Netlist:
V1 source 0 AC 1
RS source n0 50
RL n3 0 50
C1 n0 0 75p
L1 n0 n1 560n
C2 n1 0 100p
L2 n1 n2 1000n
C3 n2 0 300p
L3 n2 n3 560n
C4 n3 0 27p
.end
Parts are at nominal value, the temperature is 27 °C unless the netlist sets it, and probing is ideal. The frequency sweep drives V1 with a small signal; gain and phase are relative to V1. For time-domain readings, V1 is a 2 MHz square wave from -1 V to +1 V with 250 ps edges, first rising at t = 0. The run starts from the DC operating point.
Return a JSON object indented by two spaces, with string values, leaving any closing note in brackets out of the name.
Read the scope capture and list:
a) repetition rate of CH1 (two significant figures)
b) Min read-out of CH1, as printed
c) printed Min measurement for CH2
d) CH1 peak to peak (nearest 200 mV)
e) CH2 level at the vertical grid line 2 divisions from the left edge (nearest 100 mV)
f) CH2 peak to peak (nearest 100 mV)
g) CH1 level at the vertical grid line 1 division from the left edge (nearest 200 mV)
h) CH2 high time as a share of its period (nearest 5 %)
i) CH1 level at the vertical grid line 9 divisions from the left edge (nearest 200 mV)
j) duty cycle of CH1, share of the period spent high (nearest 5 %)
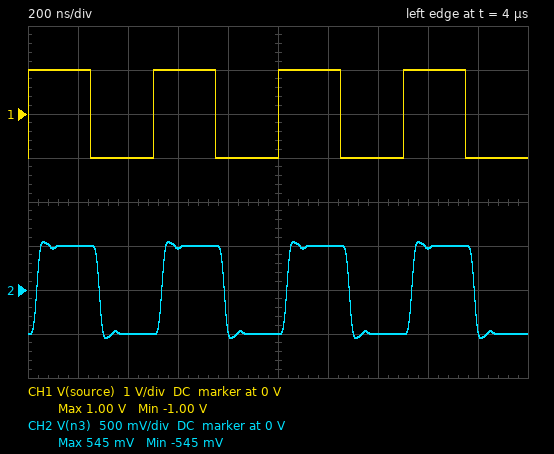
{
  "repetition rate of CH1": "2.0 MHz",
  "Min read-out of CH1, as printed": "-1.00 V",
  "printed Min measurement for CH2": "-545 mV",
  "CH1 peak to peak": "2.0 V",
  "CH2 level at the vertical grid line 2 divisions from the left edge": "-500 mV",
  "CH2 peak to peak": "1.1 V",
  "CH1 level at the vertical grid line 1 division from the left edge": "1.0 V",
  "CH2 high time as a share of its period": "50 %",
  "CH1 level at the vertical grid line 9 divisions from the left edge": "-1.0 V",
  "duty cycle of CH1, share of the period spent high": "50 %"
}
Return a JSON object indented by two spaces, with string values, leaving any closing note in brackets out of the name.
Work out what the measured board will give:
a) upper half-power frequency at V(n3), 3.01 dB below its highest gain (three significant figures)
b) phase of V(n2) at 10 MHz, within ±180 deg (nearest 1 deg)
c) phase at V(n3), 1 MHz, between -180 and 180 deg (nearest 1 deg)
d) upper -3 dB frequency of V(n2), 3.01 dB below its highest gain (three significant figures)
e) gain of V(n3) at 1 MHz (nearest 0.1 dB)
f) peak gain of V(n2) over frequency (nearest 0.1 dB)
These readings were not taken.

{
  "upper half-power frequency at V(n3), 3.01 dB below its highest gain": "15.3 MHz",
  "phase of V(n2) at 10 MHz, within ±180 deg": "-87 deg",
  "phase at V(n3), 1 MHz, between -180 and 180 deg": "-12 deg",
  "upper -3 dB frequency of V(n2), 3.01 dB below its highest gain": "18.4 MHz",
  "gain of V(n3) at 1 MHz": "-6.0 dB",
  "peak gain of V(n2) over frequency": "-5.1 dB"
}
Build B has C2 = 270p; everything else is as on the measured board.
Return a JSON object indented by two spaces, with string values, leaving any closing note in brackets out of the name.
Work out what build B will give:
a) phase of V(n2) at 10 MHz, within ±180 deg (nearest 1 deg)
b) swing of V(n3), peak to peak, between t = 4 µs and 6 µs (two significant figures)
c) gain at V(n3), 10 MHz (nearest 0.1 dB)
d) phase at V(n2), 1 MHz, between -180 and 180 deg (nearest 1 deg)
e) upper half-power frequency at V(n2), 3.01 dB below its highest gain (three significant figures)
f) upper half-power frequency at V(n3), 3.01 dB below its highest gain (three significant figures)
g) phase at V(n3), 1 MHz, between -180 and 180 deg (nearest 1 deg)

{
  "phase of V(n2) at 10 MHz, within ±180 deg": "-105 deg",
  "swing of V(n3), peak to peak, between t = 4 µs and 6 µs": "1.3 V",
  "gain at V(n3), 10 MHz": "-6.0 dB",
  "phase at V(n2), 1 MHz, between -180 and 180 deg": "-10 deg",
  "upper half-power frequency at V(n2), 3.01 dB below its highest gain": "18.6 MHz",
  "upper half-power frequency at V(n3), 3.01 dB below its highest gain": "17.9 MHz",
  "phase at V(n3), 1 MHz, between -180 and 180 deg": "-14 deg"
}
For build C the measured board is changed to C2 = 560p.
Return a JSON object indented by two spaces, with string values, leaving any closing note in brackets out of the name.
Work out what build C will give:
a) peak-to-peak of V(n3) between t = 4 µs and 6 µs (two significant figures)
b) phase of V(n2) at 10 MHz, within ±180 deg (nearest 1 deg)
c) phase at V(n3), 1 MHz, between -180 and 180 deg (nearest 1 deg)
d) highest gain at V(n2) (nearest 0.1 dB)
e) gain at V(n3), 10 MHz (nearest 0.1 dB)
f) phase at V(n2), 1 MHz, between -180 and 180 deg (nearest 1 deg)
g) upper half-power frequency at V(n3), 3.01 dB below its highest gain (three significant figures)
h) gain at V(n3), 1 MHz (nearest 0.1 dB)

{
  "peak-to-peak of V(n3) between t = 4 µs and 6 µs": "1.2 V",
  "phase of V(n2) at 10 MHz, within ±180 deg": "-136 deg",
  "phase at V(n3), 1 MHz, between -180 and 180 deg": "-16 deg",
  "highest gain at V(n2)": "-5.7 dB",
  "gain at V(n3), 10 MHz": "-7.1 dB",
  "phase at V(n2), 1 MHz, between -180 and 180 deg": "-12 deg",
  "upper half-power frequency at V(n3), 3.01 dB below its highest gain": "13.9 MHz",
  "gain at V(n3), 1 MHz": "-6.0 dB"
}
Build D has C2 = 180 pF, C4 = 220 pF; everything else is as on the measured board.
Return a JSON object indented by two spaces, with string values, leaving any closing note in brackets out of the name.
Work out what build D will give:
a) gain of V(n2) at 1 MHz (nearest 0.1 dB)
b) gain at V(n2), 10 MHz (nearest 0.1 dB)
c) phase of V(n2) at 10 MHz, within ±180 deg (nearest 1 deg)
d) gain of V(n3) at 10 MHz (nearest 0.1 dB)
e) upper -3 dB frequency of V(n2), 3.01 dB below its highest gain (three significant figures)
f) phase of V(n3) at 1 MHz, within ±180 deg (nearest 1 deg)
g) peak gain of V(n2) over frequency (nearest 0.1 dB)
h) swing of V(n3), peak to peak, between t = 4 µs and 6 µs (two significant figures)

{
  "gain of V(n2) at 1 MHz": "-6.0 dB",
  "gain at V(n2), 10 MHz": "-8.3 dB",
  "phase of V(n2) at 10 MHz, within ±180 deg": "-94 deg",
  "gain of V(n3) at 10 MHz": "-7.1 dB",
  "upper -3 dB frequency of V(n2), 3.01 dB below its highest gain": "22.5 MHz",
  "phase of V(n3) at 1 MHz, within ±180 deg": "-15 deg",
  "peak gain of V(n2) over frequency": "-3.1 dB",
  "swing of V(n3), peak to peak, between t = 4 µs and 6 µs": "1.2 V"
}
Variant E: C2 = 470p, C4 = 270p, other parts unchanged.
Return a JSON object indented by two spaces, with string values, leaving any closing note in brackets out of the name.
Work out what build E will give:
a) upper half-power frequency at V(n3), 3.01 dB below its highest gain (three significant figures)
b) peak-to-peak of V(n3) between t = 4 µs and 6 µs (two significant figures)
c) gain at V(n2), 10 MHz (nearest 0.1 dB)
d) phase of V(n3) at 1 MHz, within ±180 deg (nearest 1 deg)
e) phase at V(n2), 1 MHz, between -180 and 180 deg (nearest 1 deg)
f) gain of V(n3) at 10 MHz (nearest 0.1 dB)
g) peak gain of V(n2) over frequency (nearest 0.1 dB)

{
  "upper half-power frequency at V(n3), 3.01 dB below its highest gain": "12.3 MHz",
  "peak-to-peak of V(n3) between t = 4 µs and 6 µs": "1.2 V",
  "gain at V(n2), 10 MHz": "-8.8 dB",
  "phase of V(n3) at 1 MHz, within ±180 deg": "-18 deg",
  "phase at V(n2), 1 MHz, between -180 and 180 deg": "-14 deg",
  "gain of V(n3) at 10 MHz": "-7.0 dB",
  "peak gain of V(n2) over frequency": "-6.0 dB"
}
